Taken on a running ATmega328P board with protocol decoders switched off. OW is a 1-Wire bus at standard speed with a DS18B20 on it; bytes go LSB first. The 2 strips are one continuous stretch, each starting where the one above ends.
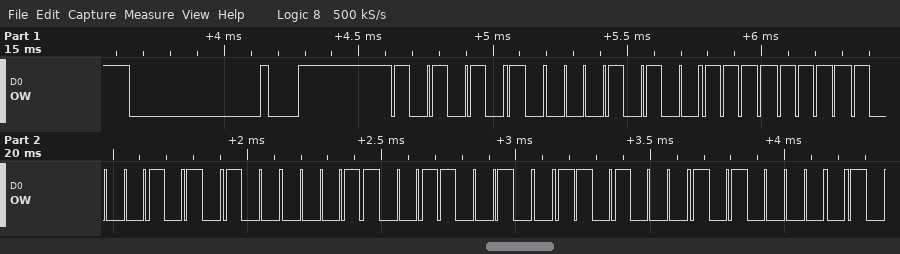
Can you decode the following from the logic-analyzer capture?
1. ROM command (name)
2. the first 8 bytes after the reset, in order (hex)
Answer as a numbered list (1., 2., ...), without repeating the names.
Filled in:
1. Match ROM
2. 55 28 FF 51 C1 4C 16 05
